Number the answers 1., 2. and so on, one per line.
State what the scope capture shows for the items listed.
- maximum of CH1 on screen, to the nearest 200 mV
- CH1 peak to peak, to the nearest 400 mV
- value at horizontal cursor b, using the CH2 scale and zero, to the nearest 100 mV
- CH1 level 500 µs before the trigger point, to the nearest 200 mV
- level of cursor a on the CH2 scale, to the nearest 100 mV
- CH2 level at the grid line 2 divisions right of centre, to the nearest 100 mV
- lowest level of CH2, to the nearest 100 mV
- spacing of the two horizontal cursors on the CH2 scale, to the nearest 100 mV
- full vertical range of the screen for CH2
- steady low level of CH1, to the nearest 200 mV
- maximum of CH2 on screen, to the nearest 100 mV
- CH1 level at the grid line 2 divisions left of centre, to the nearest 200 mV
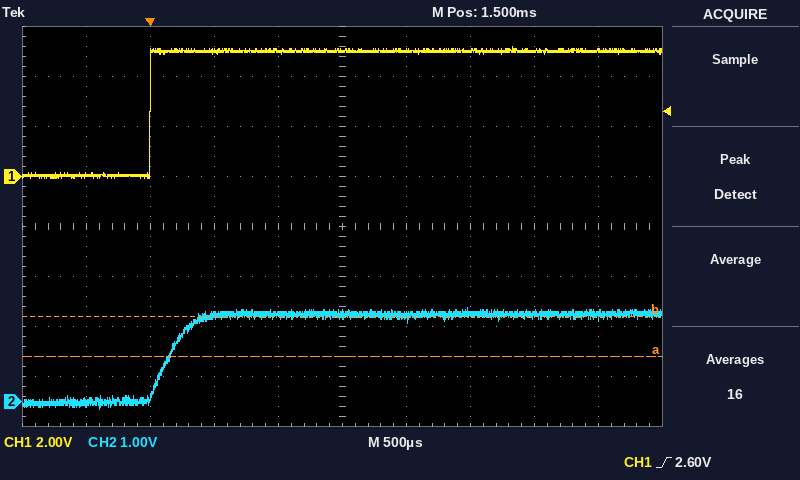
1. 5.2 V
2. 5.2 V
3. 1.7 V
4. 0.0 V
5. 900 mV
6. 1.8 V
7. -200 mV
8. 800 mV
9. 8 V
10. 0.0 V
11. 1.9 V
12. 5.0 V
